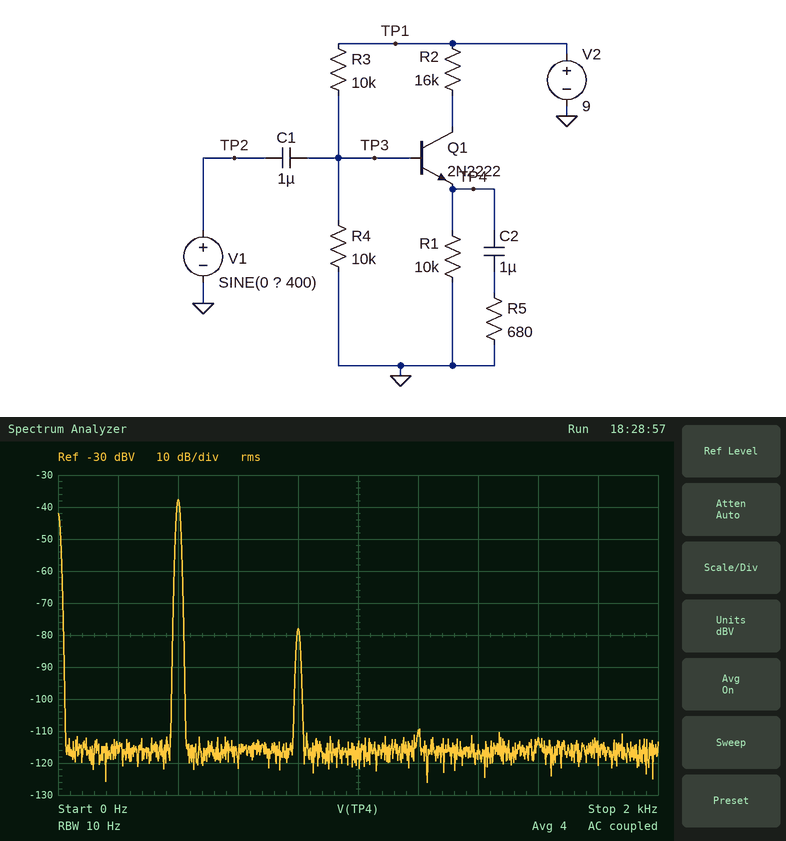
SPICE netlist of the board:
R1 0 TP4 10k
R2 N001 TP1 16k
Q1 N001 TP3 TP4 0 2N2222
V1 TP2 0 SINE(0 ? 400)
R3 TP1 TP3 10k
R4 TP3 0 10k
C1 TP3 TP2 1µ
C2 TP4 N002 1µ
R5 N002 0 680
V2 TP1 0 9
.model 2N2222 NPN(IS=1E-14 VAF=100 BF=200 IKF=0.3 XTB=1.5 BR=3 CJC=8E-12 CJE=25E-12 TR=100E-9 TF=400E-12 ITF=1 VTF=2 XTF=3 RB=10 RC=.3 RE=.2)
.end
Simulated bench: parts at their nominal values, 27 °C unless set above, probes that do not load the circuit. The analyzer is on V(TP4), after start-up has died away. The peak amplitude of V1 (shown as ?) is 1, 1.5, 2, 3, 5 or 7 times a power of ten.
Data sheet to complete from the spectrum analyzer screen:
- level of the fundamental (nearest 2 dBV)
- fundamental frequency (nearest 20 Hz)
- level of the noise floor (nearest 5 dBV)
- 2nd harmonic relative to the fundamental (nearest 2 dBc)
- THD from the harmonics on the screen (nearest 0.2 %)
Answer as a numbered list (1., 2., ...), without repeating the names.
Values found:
1. -38 dBV
2. 400 Hz
3. -115 dBV
4. -40 dBc
5. 1.0 %
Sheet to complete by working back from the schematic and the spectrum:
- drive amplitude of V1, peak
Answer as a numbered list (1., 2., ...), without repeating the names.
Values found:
1. 30 mV
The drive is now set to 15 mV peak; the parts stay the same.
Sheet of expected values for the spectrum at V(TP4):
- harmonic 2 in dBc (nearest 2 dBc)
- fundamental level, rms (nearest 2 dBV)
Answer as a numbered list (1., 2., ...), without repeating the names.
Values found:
1. -46 dBc
2. -44 dBV
